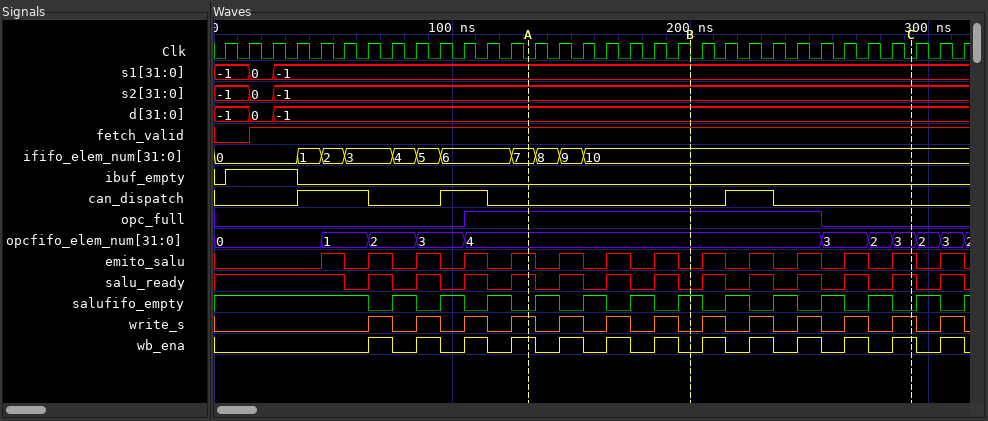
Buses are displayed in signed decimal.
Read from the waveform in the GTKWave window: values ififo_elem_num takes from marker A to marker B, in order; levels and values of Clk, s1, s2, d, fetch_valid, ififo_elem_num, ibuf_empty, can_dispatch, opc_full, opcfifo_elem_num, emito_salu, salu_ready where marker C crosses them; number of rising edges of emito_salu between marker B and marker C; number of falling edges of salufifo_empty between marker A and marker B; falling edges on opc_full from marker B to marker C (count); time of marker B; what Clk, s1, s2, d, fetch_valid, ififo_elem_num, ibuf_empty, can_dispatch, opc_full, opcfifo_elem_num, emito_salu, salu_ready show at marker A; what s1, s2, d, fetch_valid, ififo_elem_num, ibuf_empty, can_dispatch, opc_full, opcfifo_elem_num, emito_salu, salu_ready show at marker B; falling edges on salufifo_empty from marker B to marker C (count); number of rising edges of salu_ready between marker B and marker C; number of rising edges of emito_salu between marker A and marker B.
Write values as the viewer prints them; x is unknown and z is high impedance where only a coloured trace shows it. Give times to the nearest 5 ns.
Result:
7, 8, 9, 10
Clk=0, s1=-1, s2=-1, d=-1, fetch_valid=1, ififo_elem_num=10, ibuf_empty=0, can_dispatch=0, opc_full=0, opcfifo_elem_num=3, emito_salu=1, salu_ready=1
5
3
1
200 ns
Clk=0, s1=-1, s2=-1, d=-1, fetch_valid=1, ififo_elem_num=7, ibuf_empty=0, can_dispatch=0, opc_full=1, opcfifo_elem_num=4, emito_salu=1, salu_ready=1
s1=-1, s2=-1, d=-1, fetch_valid=1, ififo_elem_num=10, ibuf_empty=0, can_dispatch=0, opc_full=1, opcfifo_elem_num=4, emito_salu=0, salu_ready=0
5
5
3
